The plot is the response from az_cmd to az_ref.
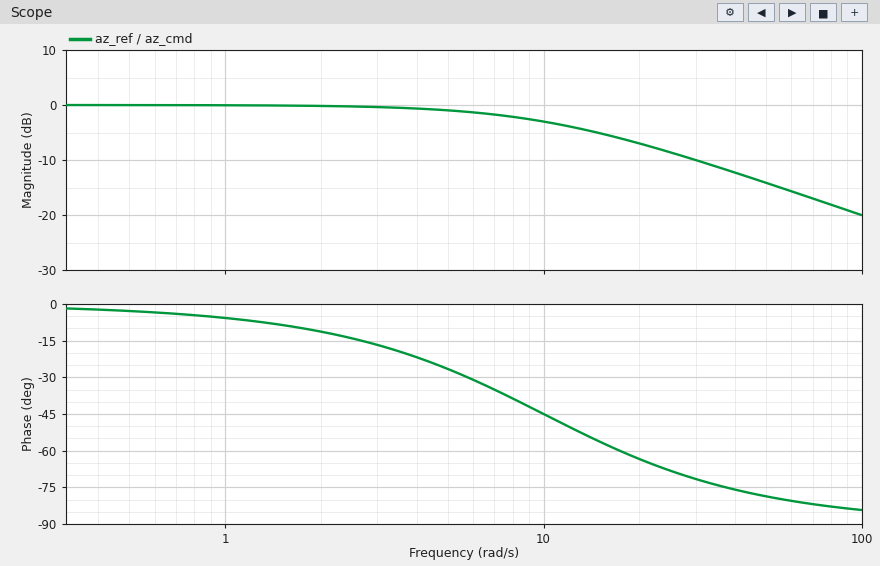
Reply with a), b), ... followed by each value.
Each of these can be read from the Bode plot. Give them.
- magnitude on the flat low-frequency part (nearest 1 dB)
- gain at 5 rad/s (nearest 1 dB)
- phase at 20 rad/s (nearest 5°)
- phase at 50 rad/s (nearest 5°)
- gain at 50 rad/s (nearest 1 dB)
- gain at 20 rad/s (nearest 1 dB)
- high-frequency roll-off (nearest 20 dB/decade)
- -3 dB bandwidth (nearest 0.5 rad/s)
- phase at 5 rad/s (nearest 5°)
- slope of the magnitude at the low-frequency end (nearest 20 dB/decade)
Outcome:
a) 0 dB
b) -1 dB
c) -65°
d) -80°
e) -14 dB
f) -7 dB
g) -20 dB/decade
h) 10.0 rad/s
i) -25°
j) 0 dB/decade
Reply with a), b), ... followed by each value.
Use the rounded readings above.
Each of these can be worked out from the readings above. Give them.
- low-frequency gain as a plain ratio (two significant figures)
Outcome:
a) 1.0
